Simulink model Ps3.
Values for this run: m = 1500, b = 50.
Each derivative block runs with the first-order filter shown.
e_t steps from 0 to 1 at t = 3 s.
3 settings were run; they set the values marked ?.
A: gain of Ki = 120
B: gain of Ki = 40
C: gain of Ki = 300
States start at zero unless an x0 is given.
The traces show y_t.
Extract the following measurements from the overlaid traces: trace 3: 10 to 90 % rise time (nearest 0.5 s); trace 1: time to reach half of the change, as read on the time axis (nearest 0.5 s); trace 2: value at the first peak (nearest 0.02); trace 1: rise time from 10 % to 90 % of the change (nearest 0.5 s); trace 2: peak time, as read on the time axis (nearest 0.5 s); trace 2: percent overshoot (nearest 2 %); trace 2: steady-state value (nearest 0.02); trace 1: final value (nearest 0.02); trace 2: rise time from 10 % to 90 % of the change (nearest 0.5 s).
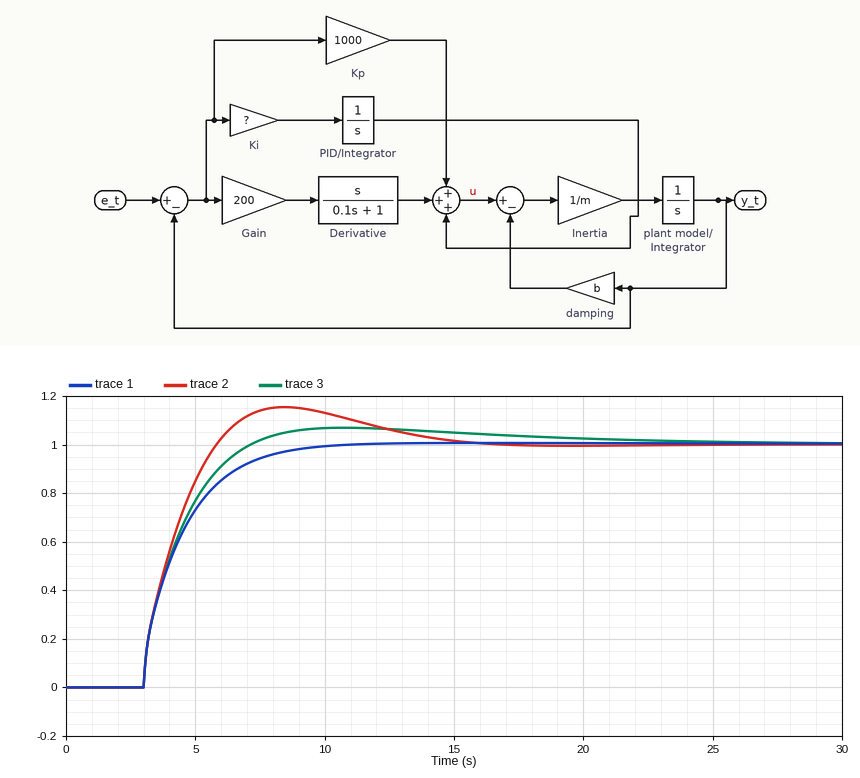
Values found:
3.0 s
4.0 s
1.16
3.5 s
8.5 s
16 %
1.00
1.00
2.0 s
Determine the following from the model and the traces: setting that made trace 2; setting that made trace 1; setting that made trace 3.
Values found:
C
B
A
